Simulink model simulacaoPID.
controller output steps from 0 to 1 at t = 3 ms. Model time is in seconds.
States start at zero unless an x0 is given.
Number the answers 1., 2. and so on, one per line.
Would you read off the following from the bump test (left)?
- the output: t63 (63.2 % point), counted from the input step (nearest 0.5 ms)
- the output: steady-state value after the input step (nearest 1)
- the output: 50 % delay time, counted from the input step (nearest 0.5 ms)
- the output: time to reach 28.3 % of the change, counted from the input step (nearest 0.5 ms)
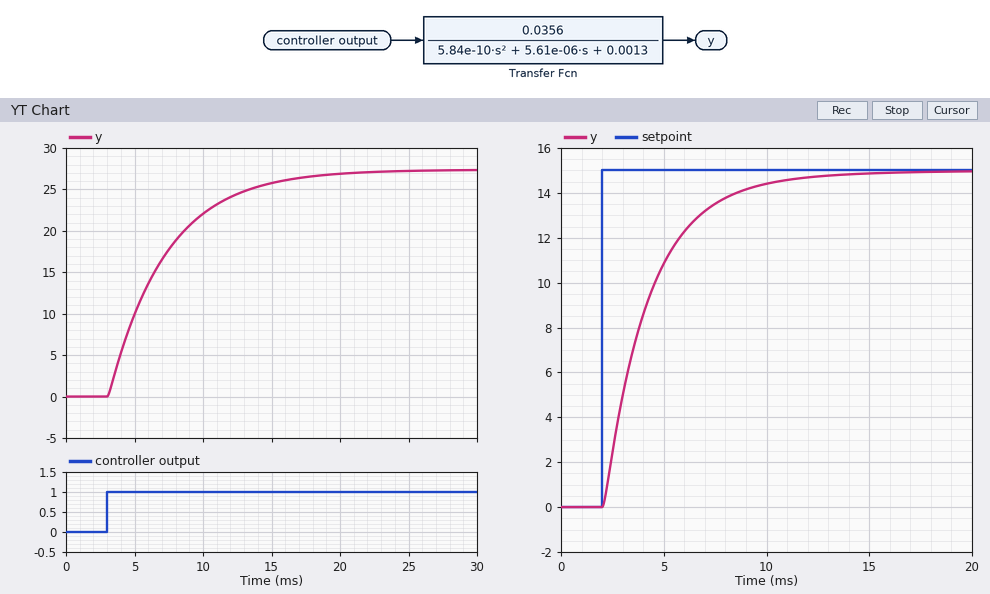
1. 4.5 ms
2. 27
3. 3.0 ms
4. 1.5 ms
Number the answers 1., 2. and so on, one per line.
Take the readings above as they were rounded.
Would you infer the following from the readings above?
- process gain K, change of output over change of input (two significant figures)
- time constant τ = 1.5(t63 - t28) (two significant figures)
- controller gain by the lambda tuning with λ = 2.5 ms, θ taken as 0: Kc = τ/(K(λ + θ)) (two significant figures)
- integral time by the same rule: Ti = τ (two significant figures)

1. 27
2. 4.5 ms
3. 0.067
4. 4.5 ms
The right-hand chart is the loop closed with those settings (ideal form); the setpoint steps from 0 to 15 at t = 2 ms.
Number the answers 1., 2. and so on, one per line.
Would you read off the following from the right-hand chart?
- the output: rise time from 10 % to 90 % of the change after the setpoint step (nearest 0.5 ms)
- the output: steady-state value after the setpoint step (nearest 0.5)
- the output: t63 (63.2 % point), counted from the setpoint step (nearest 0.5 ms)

1. 5.0 ms
2. 15.0
3. 2.5 ms
